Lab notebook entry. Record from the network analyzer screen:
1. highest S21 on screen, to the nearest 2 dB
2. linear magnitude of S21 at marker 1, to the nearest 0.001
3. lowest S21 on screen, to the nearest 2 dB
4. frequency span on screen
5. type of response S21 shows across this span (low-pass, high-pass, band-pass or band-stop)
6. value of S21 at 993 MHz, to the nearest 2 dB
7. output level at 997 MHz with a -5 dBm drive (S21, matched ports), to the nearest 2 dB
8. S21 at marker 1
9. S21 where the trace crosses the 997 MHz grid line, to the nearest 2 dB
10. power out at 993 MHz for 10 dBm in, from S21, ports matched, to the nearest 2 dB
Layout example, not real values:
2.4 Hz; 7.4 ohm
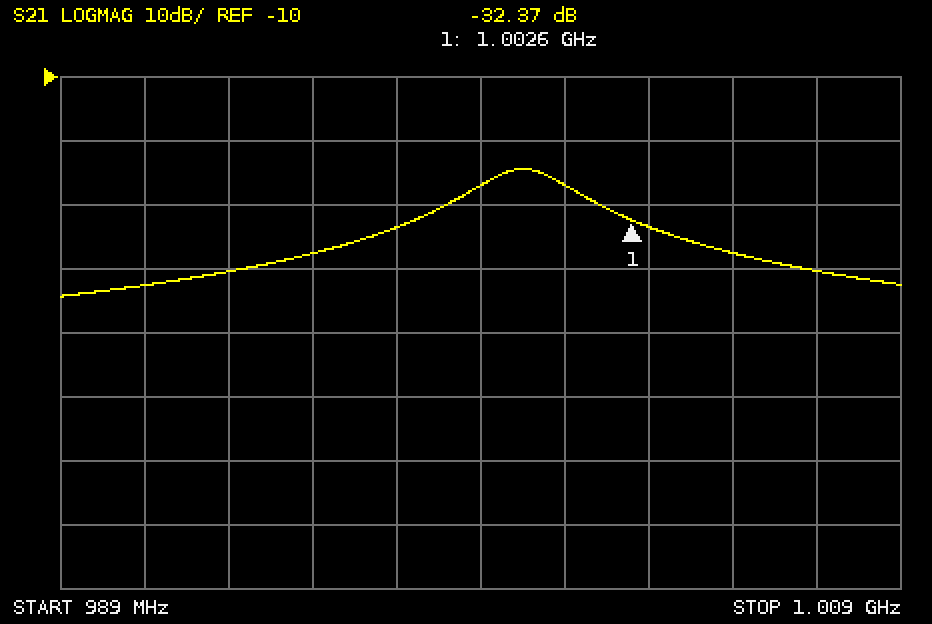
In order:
-24 dB; 0.024; -44 dB; 20 MHz; band-pass; -40 dB; -38 dBm; -32.37 dB; -34 dB; -30 dBm
